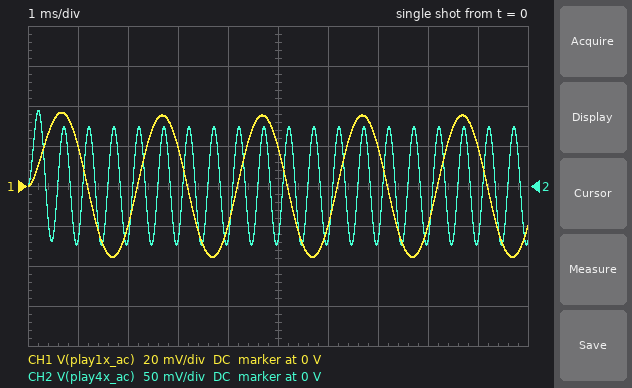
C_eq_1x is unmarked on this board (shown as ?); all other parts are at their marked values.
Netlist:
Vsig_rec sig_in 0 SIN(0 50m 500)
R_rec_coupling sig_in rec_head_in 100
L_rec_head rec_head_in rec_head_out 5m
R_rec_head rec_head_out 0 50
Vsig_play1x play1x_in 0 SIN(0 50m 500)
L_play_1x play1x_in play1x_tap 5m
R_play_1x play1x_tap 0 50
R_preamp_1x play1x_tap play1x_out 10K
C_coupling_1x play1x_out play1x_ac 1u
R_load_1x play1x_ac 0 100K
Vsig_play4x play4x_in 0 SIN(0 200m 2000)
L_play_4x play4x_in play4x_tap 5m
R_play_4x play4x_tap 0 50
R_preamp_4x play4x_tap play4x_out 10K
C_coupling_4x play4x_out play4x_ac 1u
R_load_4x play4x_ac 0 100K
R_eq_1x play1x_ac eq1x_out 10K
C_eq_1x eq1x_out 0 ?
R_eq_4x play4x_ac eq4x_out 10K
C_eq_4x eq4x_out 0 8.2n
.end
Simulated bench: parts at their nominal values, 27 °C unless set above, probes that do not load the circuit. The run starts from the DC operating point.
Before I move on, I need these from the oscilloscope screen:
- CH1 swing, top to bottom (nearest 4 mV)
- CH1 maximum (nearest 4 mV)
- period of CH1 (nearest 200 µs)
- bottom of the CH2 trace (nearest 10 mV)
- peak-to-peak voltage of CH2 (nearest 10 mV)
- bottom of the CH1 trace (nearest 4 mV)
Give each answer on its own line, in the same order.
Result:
72 mV
36 mV
2.0 ms
-70 mV
170 mV
-36 mV
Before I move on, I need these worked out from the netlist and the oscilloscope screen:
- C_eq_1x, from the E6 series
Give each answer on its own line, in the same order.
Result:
15 nF
